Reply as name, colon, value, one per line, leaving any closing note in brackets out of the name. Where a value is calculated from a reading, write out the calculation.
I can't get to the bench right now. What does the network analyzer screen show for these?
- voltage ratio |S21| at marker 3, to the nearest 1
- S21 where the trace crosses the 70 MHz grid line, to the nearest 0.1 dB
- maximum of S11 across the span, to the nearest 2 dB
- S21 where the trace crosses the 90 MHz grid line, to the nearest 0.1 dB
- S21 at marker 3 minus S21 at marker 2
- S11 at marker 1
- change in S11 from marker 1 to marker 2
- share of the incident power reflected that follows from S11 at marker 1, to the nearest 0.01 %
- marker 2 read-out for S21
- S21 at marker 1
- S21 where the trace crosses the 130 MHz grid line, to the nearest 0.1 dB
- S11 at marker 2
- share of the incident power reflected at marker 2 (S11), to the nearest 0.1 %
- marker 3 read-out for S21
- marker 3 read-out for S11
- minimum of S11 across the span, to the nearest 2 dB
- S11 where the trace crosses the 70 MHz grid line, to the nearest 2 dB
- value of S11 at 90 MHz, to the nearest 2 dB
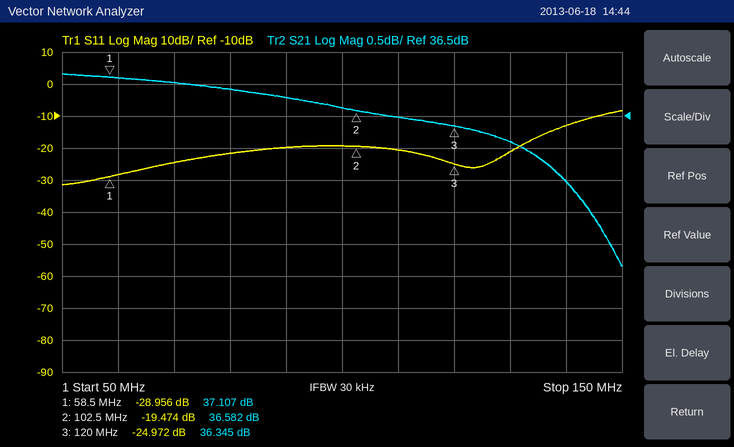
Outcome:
voltage ratio |S21| at marker 3, to the nearest 1: 10^(36.345/20) ≈ 66
S21 where the trace crosses the 70 MHz grid line, to the nearest 0.1 dB: 37.0 dB
maximum of S11 across the span, to the nearest 2 dB: -8 dB
S21 where the trace crosses the 90 MHz grid line, to the nearest 0.1 dB: 36.8 dB
S21 at marker 3 minus S21 at marker 2: 36.345 − (36.582) = -0.237 dB
S11 at marker 1: -28.956 dB
change in S11 from marker 1 to marker 2: -19.474 − (-28.956) = 9.482 dB
share of the incident power reflected that follows from S11 at marker 1, to the nearest 0.01 %: 10^(-28.956/10) ≈ 0.13 %
marker 2 read-out for S21: 36.582 dB
S21 at marker 1: 37.107 dB
S21 where the trace crosses the 130 MHz grid line, to the nearest 0.1 dB: 36.1 dB
S11 at marker 2: -19.474 dB
share of the incident power reflected at marker 2 (S11), to the nearest 0.1 %: 10^(-19.474/10) ≈ 1.1 %
marker 3 read-out for S21: 36.345 dB
marker 3 read-out for S11: -24.972 dB
minimum of S11 across the span, to the nearest 2 dB: -32 dB
S11 where the trace crosses the 70 MHz grid line, to the nearest 2 dB: -24 dB
value of S11 at 90 MHz, to the nearest 2 dB: -20 dB
